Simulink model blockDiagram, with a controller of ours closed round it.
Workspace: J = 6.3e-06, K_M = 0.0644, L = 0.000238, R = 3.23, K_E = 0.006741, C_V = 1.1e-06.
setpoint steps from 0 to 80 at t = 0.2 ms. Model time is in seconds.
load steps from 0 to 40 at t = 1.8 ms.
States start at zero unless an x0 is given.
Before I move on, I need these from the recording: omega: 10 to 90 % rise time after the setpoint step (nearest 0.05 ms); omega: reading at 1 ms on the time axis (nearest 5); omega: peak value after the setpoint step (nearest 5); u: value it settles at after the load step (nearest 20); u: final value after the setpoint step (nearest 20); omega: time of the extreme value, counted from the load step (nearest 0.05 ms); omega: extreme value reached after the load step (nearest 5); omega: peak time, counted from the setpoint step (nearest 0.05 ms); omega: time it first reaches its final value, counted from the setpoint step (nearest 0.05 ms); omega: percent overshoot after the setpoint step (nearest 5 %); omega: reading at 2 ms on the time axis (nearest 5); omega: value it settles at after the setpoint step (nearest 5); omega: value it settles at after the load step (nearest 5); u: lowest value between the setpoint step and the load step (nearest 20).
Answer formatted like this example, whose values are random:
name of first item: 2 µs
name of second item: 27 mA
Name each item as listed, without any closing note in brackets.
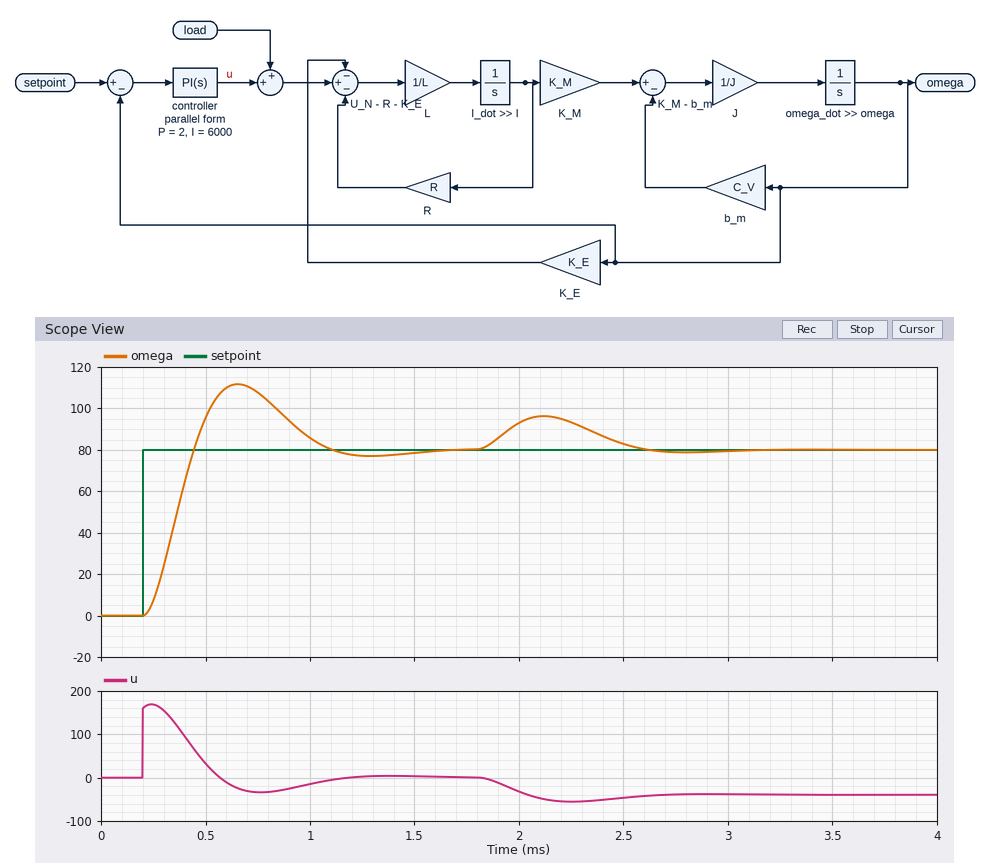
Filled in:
omega: 10 to 90 % rise time after the setpoint step: 0.15 ms
omega: reading at 1 ms on the time axis: 85
omega: peak value after the setpoint step: 110
u: value it settles at after the load step: -40
u: final value after the setpoint step: 0
omega: time of the extreme value, counted from the load step: 0.30 ms
omega: extreme value reached after the load step: 95
omega: peak time, counted from the setpoint step: 0.45 ms
omega: time it first reaches its final value, counted from the setpoint step: 0.25 ms
omega: percent overshoot after the setpoint step: 40 %
omega: reading at 2 ms on the time axis: 95
omega: value it settles at after the setpoint step: 80
omega: value it settles at after the load step: 80
u: lowest value between the setpoint step and the load step: -40
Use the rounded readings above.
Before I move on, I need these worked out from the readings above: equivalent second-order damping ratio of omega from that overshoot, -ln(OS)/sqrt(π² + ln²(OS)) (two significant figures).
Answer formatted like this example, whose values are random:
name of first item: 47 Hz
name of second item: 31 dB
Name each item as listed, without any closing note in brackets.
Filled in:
equivalent second-order damping ratio of omega from that overshoot, -ln(OS)/sqrt(π² + ln²(OS)): 0.28
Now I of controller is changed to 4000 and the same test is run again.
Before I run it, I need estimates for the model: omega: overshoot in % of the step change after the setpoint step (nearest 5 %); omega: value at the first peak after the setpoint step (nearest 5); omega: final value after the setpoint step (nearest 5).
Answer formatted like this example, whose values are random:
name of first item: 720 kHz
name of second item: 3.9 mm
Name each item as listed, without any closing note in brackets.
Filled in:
omega: overshoot in % of the step change after the setpoint step: 30 %
omega: value at the first peak after the setpoint step: 105
omega: final value after the setpoint step: 80
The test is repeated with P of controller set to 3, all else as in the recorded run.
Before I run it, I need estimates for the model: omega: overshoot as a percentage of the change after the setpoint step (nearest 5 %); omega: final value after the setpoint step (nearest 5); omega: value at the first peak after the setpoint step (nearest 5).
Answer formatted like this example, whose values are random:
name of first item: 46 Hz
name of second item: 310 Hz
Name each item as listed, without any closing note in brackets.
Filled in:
omega: overshoot as a percentage of the change after the setpoint step: 30 %
omega: final value after the setpoint step: 80
omega: value at the first peak after the setpoint step: 105
